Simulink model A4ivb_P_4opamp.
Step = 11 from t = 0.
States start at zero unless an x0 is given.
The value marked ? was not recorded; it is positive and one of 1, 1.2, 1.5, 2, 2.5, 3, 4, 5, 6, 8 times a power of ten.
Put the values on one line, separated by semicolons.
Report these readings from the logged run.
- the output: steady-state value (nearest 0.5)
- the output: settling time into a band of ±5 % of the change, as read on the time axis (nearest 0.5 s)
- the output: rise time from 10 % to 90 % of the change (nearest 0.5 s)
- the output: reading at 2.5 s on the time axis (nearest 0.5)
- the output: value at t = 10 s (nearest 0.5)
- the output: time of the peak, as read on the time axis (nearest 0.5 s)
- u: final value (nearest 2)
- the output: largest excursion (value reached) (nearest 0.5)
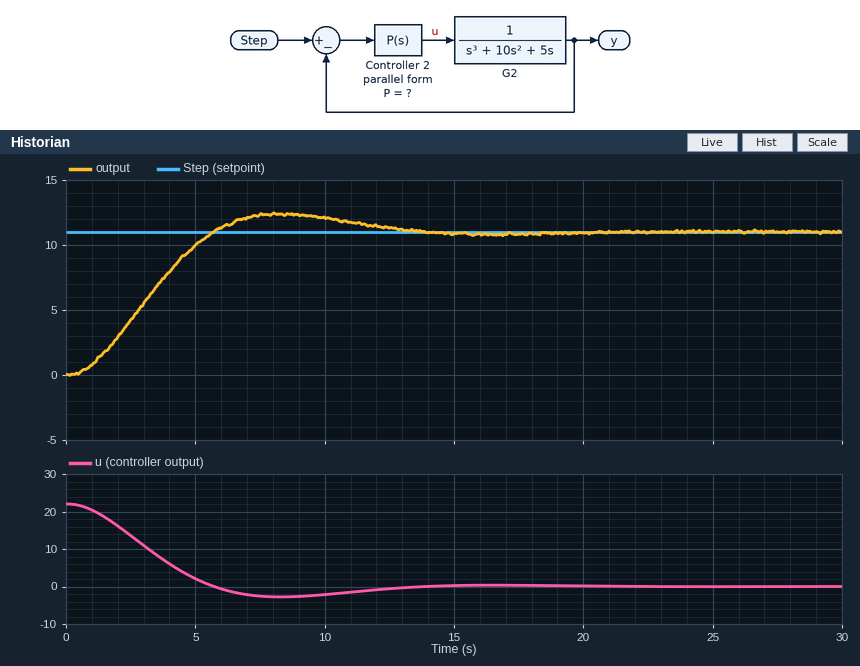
11.0; 11.5 s; 4.0 s; 4.0; 12.0; 8.5 s; 0; 12.5
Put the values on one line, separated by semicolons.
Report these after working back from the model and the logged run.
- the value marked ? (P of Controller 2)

2
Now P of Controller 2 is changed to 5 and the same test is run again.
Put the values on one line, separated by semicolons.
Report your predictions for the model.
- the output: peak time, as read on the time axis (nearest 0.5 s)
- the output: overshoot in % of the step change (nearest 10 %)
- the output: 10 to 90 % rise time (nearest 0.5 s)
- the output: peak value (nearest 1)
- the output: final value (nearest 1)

4.5 s; 30 %; 2.0 s; 15; 11
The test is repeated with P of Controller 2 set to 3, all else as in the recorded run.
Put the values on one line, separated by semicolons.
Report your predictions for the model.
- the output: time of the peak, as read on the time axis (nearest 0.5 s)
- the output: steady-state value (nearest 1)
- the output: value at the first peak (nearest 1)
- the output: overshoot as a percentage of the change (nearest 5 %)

6.5 s; 11; 13; 20 %
